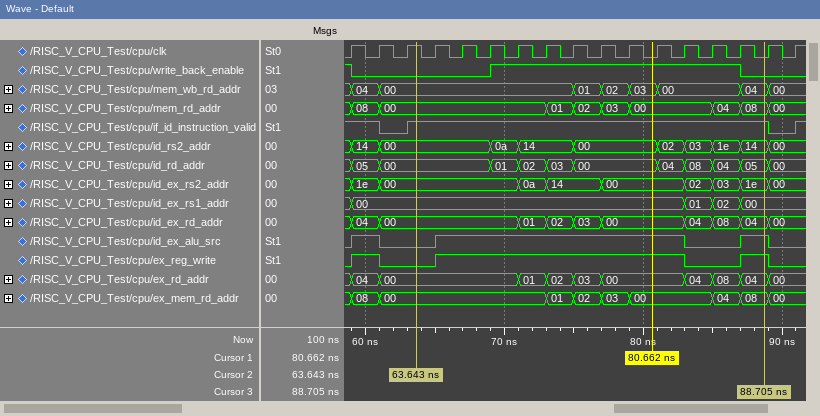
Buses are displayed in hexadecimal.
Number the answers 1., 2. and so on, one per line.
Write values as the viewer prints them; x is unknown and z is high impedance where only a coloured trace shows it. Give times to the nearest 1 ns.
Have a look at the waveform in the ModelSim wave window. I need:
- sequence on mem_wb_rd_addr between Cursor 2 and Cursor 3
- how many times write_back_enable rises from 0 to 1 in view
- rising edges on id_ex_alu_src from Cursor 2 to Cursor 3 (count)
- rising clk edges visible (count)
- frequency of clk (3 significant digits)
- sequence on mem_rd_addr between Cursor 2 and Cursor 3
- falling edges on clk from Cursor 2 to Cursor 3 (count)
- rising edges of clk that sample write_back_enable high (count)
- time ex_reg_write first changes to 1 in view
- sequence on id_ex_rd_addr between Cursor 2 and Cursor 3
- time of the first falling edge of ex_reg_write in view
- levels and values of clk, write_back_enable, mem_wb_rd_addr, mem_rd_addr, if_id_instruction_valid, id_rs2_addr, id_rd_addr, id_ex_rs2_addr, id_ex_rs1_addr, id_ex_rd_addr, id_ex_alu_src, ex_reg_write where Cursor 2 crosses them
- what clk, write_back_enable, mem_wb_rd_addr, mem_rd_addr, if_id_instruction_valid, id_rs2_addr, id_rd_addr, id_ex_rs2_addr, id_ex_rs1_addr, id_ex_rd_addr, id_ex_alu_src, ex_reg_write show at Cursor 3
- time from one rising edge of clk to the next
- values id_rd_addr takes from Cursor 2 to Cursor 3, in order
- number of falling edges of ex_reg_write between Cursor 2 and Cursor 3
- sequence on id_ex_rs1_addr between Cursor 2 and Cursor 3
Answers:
1. 00, 01, 02, 03, 00, 04
2. 1
3. 2
4. 17
5. 500 MHz
6. 00, 01, 02, 03, 00, 04, 08
7. 13
8. 10
9. 59 ns
10. 00, 01, 02, 03, 00, 04, 08, 04
11. 61 ns
12. clk=1, write_back_enable=0, mem_wb_rd_addr=00, mem_rd_addr=00, if_id_instruction_valid=1, id_rs2_addr=00, id_rd_addr=00, id_ex_rs2_addr=00, id_ex_rs1_addr=00, id_ex_rd_addr=00, id_ex_alu_src=0, ex_reg_write=0
13. clk=0, write_back_enable=0, mem_wb_rd_addr=04, mem_rd_addr=08, if_id_instruction_valid=1, id_rs2_addr=14, id_rd_addr=05, id_ex_rs2_addr=1e, id_ex_rs1_addr=00, id_ex_rd_addr=04, id_ex_alu_src=1, ex_reg_write=1
14. 2 ns
15. 00, 01, 02, 03, 00, 04, 08, 04, 05
16. 1
17. 00, 01, 02, 00
